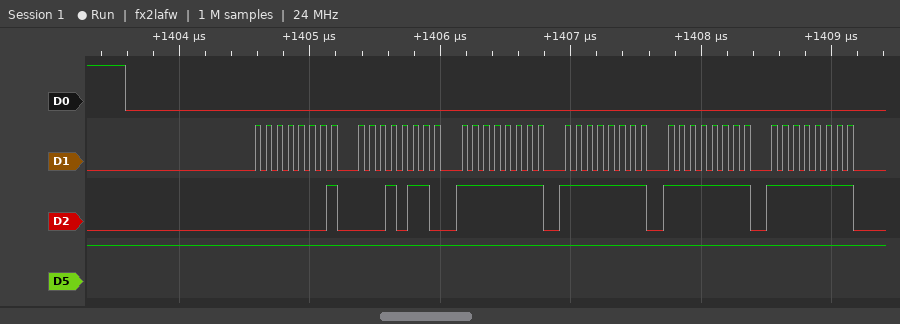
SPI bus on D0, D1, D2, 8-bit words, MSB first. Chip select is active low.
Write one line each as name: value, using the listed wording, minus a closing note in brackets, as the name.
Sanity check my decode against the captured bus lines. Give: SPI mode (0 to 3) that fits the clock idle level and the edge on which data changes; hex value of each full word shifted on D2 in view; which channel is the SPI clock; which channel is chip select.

SPI mode (0 to 3) that fits the clock idle level and the edge on which data changes: 0
hex value of each full word shifted on D2 in view: 01, 16, FF, FF, FF, FF
which channel is the SPI clock: D1
which channel is chip select: D0
